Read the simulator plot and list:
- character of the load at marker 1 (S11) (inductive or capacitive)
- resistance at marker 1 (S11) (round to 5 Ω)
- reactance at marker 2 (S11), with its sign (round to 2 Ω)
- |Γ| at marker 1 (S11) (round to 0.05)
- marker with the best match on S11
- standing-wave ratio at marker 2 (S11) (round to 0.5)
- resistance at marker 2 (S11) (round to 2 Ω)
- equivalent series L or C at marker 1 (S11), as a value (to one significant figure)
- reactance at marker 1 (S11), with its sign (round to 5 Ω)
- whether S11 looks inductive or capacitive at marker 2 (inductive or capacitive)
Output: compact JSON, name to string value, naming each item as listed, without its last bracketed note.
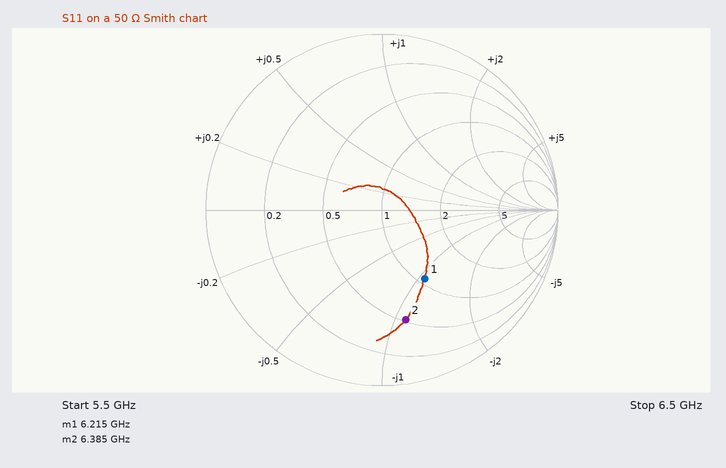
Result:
{"character of the load at marker 1 (S11)": "capacitive", "resistance at marker 1 (S11)": "55 Ω", "reactance at marker 2 (S11), with its sign": "-54 Ω", "|Γ| at marker 1 (S11)": "0.45", "marker with the best match on S11": "marker 1", "standing-wave ratio at marker 2 (S11)": "4.5", "resistance at marker 2 (S11)": "26 Ω", "equivalent series L or C at marker 1 (S11), as a value": "500 fF", "reactance at marker 1 (S11), with its sign": "-55 Ω", "whether S11 looks inductive or capacitive at marker 2": "capacitive"}
